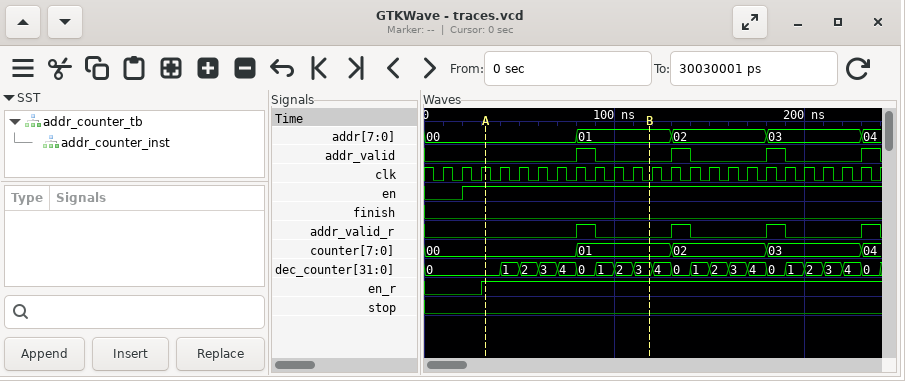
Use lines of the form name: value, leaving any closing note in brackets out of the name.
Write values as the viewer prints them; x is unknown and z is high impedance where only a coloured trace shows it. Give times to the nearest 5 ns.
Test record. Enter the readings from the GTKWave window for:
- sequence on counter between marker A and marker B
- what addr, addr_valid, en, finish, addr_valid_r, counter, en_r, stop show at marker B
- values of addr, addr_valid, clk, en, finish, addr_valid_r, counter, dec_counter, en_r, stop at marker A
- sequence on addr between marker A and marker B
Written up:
sequence on counter between marker A and marker B: 00, 01
what addr, addr_valid, en, finish, addr_valid_r, counter, en_r, stop show at marker B: addr=01, addr_valid=0, en=1, finish=0, addr_valid_r=0, counter=01, en_r=1, stop=0
values of addr, addr_valid, clk, en, finish, addr_valid_r, counter, dec_counter, en_r, stop at marker A: addr=00, addr_valid=0, clk=1, en=1, finish=0, addr_valid_r=0, counter=00, dec_counter=0, en_r=1, stop=0
sequence on addr between marker A and marker B: 00, 01
